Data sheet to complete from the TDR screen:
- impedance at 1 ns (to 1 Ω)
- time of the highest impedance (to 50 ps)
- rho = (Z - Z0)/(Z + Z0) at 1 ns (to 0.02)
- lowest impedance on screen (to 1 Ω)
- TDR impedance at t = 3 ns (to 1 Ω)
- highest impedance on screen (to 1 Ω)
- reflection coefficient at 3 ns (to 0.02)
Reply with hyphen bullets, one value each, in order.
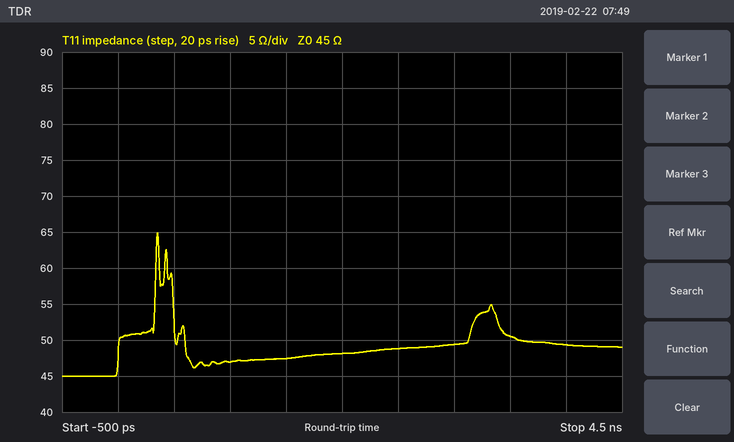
- 47 Ω
- 350 ps
- +0.02
- 45 Ω
- 49 Ω
- 65 Ω
- +0.04
